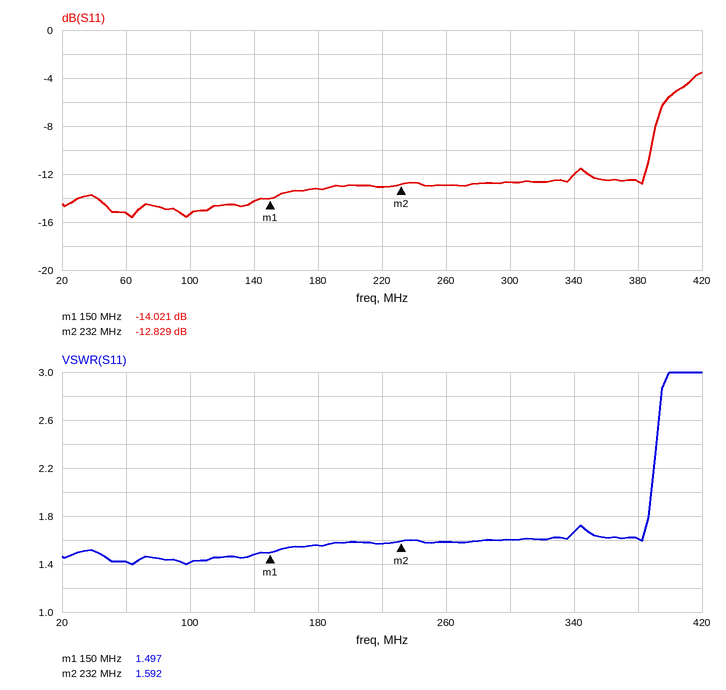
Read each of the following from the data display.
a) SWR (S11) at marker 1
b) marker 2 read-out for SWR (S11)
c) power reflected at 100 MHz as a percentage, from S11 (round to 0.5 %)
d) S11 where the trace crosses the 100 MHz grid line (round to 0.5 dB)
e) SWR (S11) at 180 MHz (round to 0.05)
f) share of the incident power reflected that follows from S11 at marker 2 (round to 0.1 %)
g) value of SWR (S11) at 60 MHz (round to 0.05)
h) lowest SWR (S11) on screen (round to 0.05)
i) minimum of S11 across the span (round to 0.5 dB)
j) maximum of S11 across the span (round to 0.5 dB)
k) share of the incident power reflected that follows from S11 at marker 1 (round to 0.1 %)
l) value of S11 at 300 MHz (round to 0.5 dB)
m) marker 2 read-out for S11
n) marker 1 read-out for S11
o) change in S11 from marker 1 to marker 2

1.497
1.592
3.0 %
-15.5 dB
1.55
5.2 %
1.40
1.40
-15.5 dB
-3.5 dB
4.0 %
-12.5 dB
-12.829 dB
-14.021 dB
1.192 dB
